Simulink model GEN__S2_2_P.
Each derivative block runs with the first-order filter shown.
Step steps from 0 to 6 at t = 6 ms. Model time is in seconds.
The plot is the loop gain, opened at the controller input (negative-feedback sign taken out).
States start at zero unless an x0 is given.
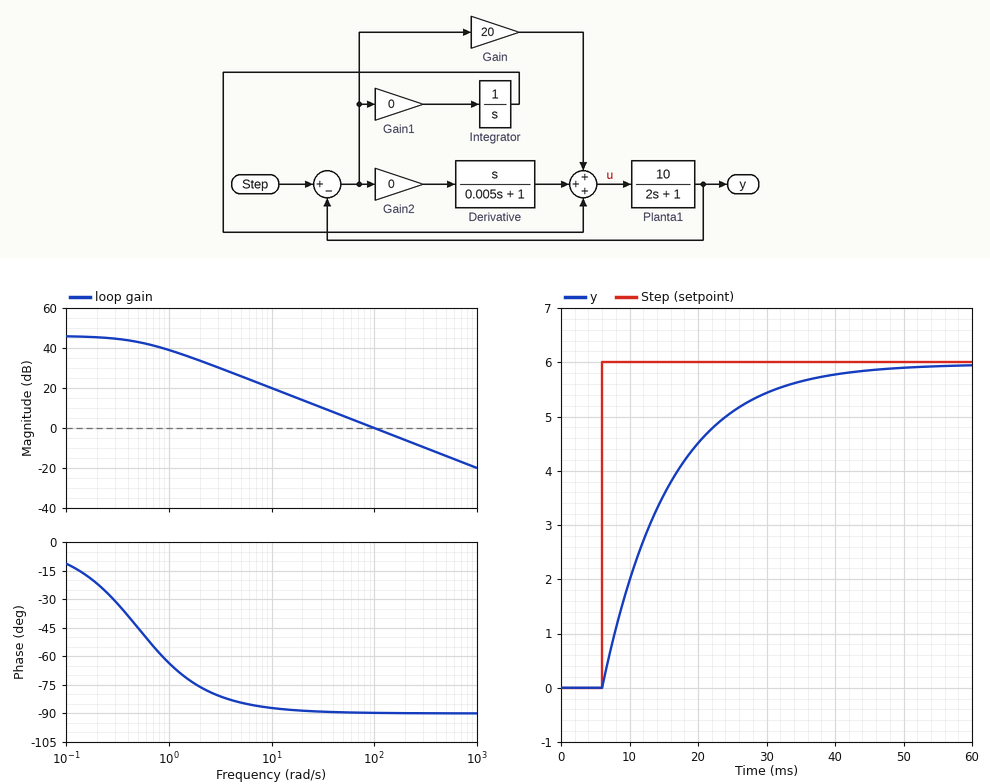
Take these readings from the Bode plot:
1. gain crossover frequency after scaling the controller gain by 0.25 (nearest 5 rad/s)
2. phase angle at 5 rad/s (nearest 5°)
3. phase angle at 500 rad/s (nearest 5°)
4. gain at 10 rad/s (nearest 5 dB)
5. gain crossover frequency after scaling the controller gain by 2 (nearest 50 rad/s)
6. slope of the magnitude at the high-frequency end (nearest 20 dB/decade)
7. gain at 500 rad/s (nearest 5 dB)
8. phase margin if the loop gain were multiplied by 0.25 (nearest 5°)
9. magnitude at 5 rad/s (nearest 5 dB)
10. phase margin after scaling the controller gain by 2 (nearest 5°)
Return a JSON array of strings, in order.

["25 rad/s", "-85°", "-90°", "20 dB", "200 rad/s", "-20 dB/decade", "-15 dB", "90°", "25 dB", "90°"]
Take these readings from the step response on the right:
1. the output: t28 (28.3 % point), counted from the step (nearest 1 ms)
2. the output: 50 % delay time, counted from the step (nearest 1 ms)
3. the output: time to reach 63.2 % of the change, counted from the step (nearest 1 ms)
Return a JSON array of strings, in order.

["3 ms", "7 ms", "10 ms"]
